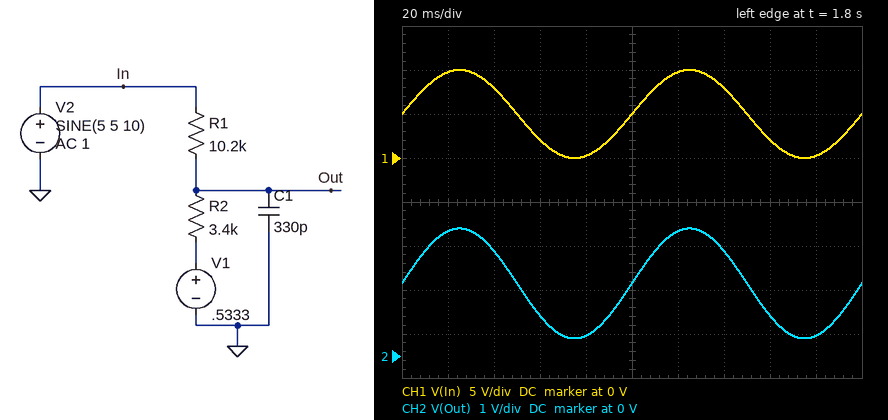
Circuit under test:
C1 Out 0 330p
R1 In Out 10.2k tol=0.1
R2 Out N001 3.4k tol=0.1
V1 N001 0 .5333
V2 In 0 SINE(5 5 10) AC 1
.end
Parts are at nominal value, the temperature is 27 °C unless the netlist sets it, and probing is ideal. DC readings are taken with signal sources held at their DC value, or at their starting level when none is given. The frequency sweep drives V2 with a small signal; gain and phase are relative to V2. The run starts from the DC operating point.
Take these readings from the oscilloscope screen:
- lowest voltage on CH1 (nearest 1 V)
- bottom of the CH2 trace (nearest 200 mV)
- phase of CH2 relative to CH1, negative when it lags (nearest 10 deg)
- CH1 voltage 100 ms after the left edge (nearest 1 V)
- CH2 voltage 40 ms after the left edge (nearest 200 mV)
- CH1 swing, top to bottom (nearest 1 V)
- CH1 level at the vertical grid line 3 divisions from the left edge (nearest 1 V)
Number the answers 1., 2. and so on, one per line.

1. 0 V
2. 400 mV
3. 0 deg
4. 5 V
5. 2.4 V
6. 10 V
7. 2 V
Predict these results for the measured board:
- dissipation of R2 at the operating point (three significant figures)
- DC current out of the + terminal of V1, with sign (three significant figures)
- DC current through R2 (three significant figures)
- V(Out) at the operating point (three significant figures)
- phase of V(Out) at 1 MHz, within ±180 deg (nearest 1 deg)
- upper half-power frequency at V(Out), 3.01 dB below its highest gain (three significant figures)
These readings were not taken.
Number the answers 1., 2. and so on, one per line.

1. 367 µW
2. -328 µA
3. 328 µA
4. 1.65 V
5. -79 deg
6. 189 kHz
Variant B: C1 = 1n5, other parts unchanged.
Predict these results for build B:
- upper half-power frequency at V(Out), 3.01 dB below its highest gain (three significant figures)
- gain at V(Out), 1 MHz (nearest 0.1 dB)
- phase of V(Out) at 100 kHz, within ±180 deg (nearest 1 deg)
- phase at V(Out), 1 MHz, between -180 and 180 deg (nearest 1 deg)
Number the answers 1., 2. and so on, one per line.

1. 41.6 kHz
2. -39.7 dB
3. -67 deg
4. -88 deg
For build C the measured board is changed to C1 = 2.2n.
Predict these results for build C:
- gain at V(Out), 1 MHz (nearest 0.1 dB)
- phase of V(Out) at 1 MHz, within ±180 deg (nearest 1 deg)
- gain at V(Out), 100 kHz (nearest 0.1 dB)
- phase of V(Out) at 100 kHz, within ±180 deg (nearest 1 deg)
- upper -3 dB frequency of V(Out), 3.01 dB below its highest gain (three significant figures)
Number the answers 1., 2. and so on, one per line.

1. -43.0 dB
2. -88 deg
3. -23.3 dB
4. -74 deg
5. 28.4 kHz
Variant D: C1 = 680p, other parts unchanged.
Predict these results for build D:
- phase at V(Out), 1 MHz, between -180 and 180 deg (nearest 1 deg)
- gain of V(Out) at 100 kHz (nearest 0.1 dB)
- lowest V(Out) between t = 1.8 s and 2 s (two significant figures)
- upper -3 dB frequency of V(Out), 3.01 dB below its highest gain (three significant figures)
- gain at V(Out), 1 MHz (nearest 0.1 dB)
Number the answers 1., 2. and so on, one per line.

1. -85 deg
2. -15.4 dB
3. 400 mV
4. 91.8 kHz
5. -32.8 dB
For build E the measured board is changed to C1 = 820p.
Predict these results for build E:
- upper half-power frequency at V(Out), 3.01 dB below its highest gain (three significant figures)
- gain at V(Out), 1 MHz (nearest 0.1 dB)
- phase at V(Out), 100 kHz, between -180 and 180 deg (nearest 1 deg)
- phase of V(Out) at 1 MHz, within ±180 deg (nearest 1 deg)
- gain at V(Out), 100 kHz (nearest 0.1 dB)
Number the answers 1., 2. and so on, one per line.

1. 76.1 kHz
2. -34.4 dB
3. -53 deg
4. -86 deg
5. -16.4 dB
